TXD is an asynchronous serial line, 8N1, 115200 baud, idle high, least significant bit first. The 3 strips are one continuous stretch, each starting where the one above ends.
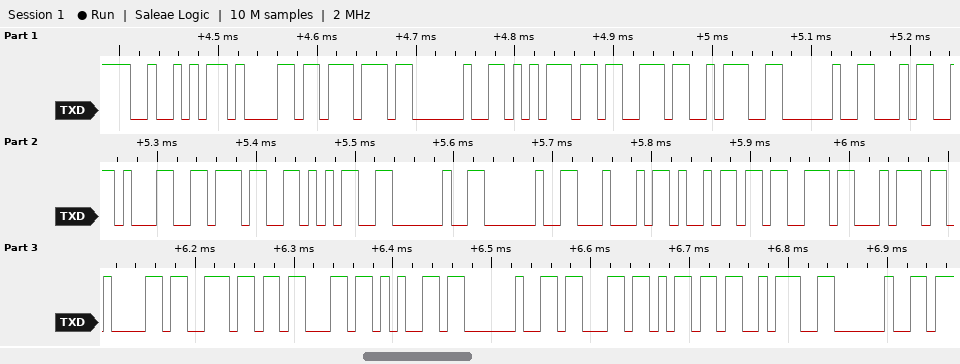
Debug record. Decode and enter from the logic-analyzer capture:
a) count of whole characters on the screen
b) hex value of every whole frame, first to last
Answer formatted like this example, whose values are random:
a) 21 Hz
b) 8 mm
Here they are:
a) 27
b) 52 61 77 20 75 73 3A 20 34 31 37 35 20 20 44 69 73 74 61 6E 63 65 20 63 6D 3A 20
